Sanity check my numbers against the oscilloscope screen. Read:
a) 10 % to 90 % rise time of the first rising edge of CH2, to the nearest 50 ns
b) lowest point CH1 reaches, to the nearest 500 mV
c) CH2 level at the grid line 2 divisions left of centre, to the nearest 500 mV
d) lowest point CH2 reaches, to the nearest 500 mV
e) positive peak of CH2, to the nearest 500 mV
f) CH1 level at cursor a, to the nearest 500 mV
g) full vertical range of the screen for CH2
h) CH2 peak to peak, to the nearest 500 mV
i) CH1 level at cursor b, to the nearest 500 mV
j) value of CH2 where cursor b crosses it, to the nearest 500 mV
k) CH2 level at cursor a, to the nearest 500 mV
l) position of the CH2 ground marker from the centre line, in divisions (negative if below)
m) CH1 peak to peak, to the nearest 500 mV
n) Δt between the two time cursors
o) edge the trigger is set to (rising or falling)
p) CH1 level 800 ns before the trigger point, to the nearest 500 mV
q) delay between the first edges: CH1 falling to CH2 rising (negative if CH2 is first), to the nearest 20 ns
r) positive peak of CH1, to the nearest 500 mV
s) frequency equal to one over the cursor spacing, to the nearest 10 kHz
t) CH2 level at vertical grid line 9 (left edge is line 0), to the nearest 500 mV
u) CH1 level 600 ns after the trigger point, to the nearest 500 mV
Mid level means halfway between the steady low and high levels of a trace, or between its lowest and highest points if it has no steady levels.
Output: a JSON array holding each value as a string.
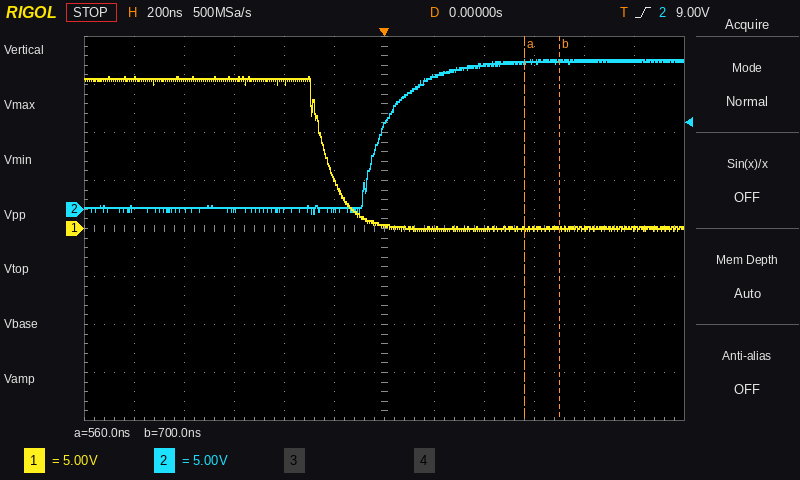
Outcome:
["300 ns", "0.0 V", "0.0 V", "-500 mV", "15.5 V", "0.0 V", "40 V", "16.0 V", "0.0 V", "15.5 V", "15.5 V", "+0.4 div", "16.0 V", "140 ns", "rising", "15.5 V", "+220 ns", "16.0 V", "7.14 MHz", "15.5 V", "0.0 V"]
